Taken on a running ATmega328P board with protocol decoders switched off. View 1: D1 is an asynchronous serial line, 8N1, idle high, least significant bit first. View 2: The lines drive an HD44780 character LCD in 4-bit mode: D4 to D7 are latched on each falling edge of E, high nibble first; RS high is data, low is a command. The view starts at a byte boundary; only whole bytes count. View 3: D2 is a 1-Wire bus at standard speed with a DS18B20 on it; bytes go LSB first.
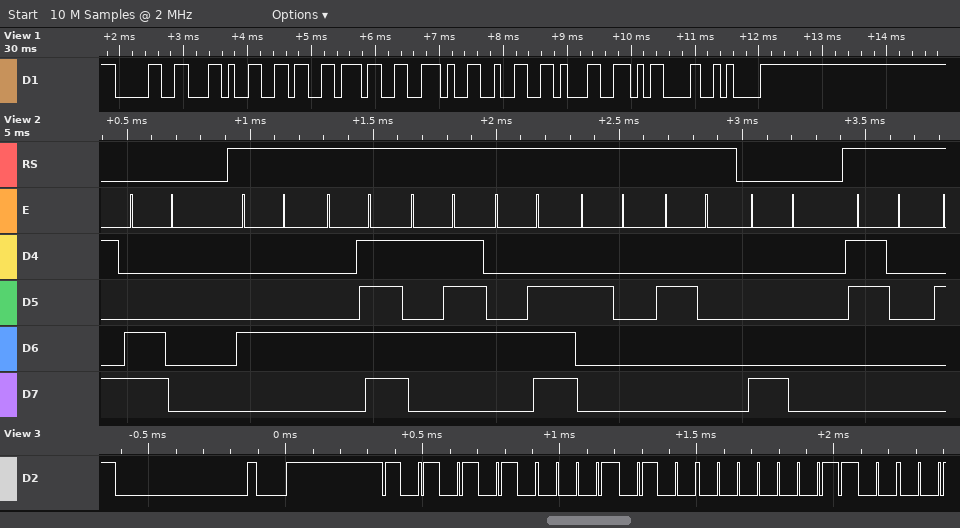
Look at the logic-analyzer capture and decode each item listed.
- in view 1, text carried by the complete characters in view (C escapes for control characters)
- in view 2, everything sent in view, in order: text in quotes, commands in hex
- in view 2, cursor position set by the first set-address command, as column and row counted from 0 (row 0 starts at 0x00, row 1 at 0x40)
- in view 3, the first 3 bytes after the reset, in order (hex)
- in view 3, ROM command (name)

"0,67.21\r\n"
0xC0 "DOWN  " 0x80 "0"
column 0, row 1
55 28 C0
Match ROM
